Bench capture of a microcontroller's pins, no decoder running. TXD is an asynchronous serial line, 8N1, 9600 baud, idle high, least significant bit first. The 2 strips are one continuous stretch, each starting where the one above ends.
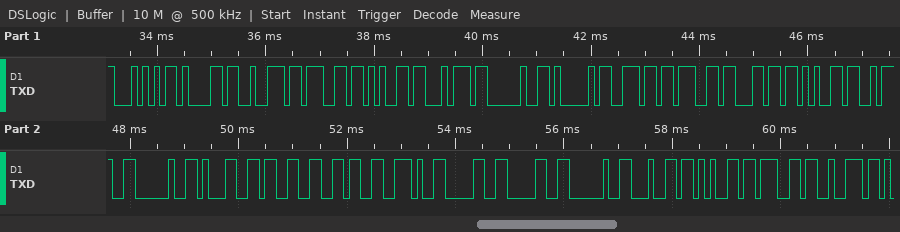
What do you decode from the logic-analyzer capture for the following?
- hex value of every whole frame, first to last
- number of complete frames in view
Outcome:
54 61 72 67 65 74 20 41 6E 67 6C 65 3A 20 31 33 36 2E 30 30 20 64 65 67 72
25
